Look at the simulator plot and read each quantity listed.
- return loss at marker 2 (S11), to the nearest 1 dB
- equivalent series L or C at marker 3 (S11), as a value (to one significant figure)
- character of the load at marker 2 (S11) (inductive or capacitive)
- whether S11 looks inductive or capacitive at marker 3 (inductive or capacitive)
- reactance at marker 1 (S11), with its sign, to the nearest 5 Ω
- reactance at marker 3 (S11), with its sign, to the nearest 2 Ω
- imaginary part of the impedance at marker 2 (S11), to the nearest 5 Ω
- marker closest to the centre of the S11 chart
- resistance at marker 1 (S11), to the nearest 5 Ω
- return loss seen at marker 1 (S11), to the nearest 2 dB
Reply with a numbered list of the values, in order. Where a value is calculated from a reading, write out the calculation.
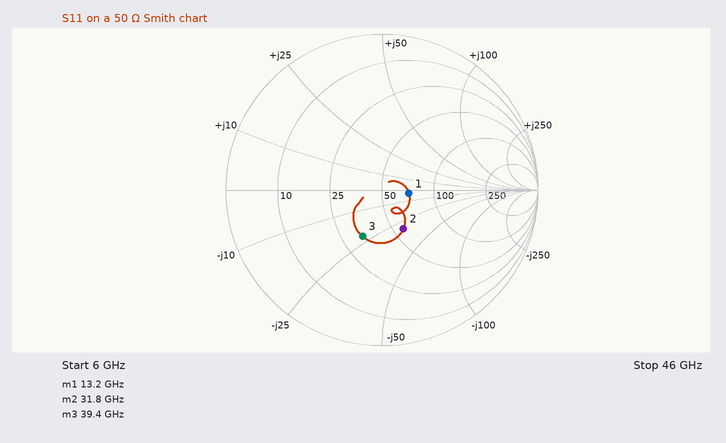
1. 11 dB
2. C = 1/(2π × 39.4 GHz × 22 Ω) ≈ 184 fF, so 200 fF to one significant figure
3. capacitive
4. capacitive
5. -5 Ω
6. -22 Ω
7. -30 Ω
8. marker 1
9. 70 Ω
10. 16 dB
